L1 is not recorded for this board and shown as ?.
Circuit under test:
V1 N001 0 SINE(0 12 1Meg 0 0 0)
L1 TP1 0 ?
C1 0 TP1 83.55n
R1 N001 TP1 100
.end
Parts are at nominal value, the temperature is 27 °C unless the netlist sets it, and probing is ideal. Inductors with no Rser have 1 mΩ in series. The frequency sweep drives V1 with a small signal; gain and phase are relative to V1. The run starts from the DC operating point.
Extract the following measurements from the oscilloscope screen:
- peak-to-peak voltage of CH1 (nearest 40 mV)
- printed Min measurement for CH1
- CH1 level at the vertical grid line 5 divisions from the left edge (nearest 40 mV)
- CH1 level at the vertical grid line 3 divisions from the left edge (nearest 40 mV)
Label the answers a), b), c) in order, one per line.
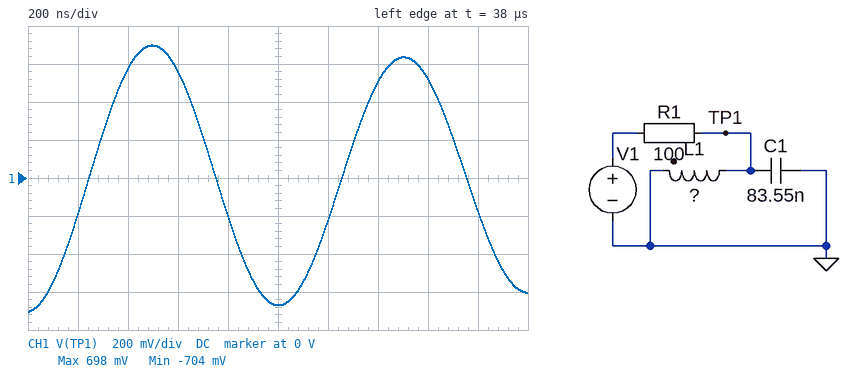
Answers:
a) 1.40 V
b) -704 mV
c) -680 mV
d) 560 mV
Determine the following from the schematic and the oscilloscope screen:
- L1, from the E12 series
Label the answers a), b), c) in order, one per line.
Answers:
a) 470 nH
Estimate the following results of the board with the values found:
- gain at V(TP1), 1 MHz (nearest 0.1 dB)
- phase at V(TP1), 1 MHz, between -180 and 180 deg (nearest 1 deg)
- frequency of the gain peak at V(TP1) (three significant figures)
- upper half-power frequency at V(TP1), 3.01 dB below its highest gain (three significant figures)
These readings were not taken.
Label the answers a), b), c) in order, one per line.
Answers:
a) -25.4 dB
b) -87 deg
c) 803 kHz
d) 813 kHz
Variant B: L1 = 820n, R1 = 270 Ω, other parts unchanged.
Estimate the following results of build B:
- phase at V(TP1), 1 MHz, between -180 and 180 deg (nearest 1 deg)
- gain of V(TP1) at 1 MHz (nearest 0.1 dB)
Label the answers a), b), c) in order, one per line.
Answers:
a) -89 deg
b) -39.0 dB
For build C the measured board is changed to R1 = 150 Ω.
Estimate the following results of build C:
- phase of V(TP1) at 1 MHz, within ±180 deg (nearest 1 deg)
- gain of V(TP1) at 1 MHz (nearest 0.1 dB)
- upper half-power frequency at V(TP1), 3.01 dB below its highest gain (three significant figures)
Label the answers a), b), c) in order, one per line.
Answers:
a) -88 deg
b) -28.9 dB
c) 810 kHz
